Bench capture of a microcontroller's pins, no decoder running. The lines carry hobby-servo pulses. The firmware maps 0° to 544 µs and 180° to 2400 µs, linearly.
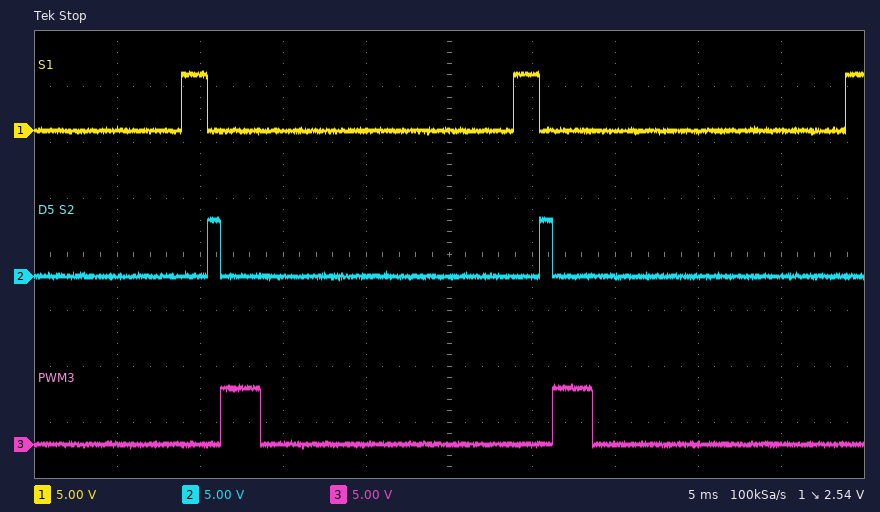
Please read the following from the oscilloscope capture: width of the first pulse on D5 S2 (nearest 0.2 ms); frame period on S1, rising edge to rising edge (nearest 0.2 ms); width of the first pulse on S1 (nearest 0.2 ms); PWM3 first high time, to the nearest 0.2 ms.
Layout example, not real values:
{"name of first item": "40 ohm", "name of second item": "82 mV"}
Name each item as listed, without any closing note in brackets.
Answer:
{"width of the first pulse on D5 S2": "0.8 ms", "frame period on S1, rising edge to rising edge": "20.0 ms", "width of the first pulse on S1": "1.6 ms", "PWM3 first high time, to the nearest 0.2 ms": "2.4 ms"}
